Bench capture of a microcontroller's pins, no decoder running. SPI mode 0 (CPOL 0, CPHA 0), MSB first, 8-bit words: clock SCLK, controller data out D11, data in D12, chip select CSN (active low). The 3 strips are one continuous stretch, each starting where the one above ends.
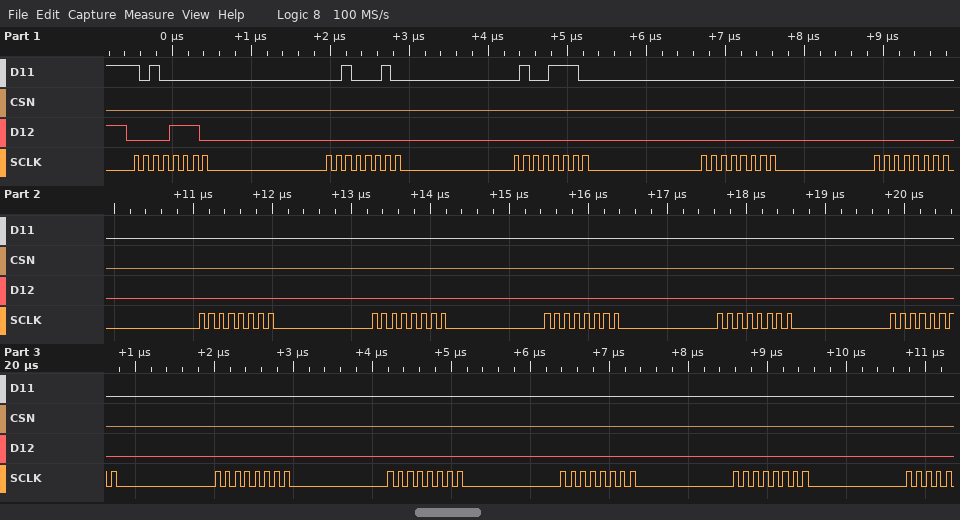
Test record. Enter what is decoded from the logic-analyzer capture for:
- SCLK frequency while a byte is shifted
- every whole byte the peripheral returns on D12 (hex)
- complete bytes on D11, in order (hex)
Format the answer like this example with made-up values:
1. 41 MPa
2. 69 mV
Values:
1. 8 MHz
2. 0E 00 00 00 00 00 00 00 00 00 00 00 00 00
3. A0 22 4E 00 00 00 00 00 00 00 00 00 00 00
